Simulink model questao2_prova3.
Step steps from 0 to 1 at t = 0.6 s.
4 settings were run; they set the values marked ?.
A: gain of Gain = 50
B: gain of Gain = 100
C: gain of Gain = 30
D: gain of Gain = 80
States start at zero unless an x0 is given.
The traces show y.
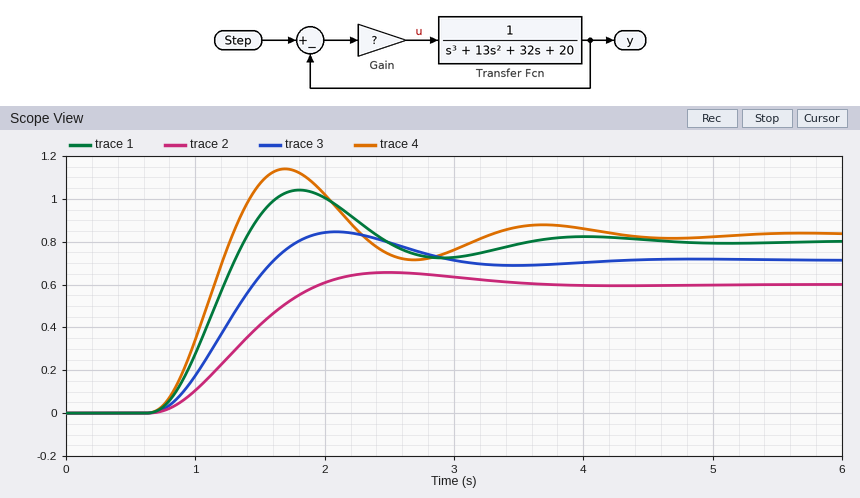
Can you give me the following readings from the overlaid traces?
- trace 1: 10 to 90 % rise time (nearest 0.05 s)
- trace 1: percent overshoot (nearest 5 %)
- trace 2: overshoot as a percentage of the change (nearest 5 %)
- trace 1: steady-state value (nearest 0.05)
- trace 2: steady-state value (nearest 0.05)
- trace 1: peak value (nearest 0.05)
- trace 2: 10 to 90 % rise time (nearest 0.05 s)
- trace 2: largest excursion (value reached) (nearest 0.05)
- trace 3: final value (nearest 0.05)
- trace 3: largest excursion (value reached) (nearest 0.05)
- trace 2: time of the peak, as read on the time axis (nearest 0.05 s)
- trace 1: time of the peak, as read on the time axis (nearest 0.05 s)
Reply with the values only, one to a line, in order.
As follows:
0.50 s
30 %
10 %
0.80
0.60
1.05
0.85 s
0.65
0.70
0.85
2.50 s
1.80 s
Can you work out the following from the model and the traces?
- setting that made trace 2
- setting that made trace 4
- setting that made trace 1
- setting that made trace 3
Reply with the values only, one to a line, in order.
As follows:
C
B
D
A
